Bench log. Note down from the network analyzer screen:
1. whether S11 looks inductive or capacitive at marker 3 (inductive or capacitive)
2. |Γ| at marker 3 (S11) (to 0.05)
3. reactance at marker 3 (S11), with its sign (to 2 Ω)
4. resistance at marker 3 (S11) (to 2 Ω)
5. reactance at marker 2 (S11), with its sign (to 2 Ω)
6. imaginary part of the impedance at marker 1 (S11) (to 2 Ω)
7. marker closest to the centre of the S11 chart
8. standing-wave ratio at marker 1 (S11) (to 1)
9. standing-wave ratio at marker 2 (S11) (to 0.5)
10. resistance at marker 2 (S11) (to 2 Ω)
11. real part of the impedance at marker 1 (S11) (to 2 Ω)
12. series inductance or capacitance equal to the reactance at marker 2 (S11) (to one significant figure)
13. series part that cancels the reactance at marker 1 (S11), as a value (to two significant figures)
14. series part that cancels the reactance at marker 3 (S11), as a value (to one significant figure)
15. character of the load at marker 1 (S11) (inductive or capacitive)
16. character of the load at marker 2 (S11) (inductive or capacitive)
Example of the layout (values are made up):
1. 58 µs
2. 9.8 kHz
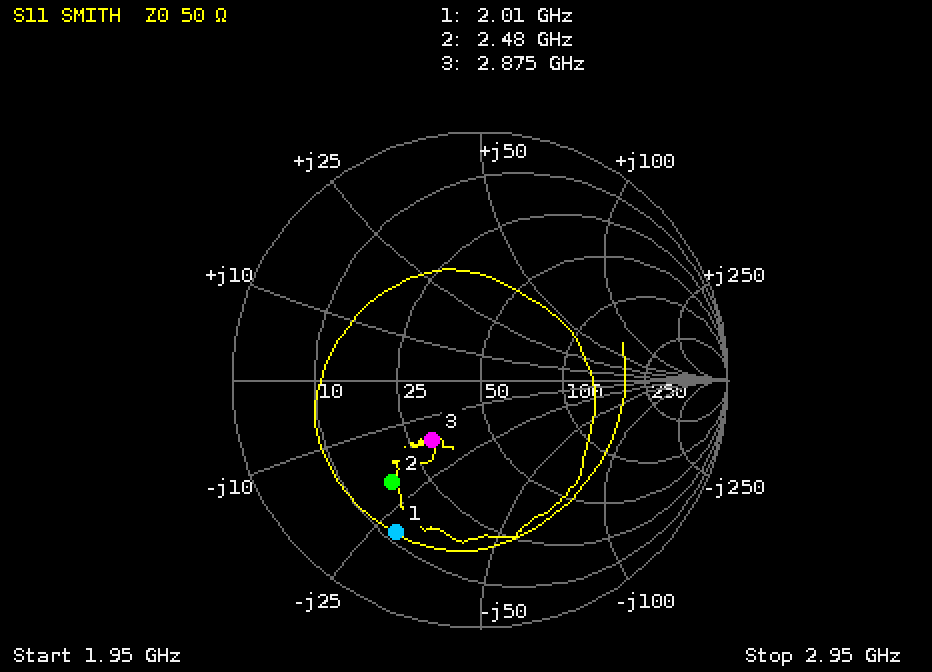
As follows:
1. capacitive
2. 0.30
3. -16 Ω
4. 30 Ω
5. -20 Ω
6. -28 Ω
7. marker 3
8. 6
9. 3.5
10. 18 Ω
11. 12 Ω
12. 3 pF
13. 2.2 nH
14. 900 pH
15. capacitive
16. capacitive
